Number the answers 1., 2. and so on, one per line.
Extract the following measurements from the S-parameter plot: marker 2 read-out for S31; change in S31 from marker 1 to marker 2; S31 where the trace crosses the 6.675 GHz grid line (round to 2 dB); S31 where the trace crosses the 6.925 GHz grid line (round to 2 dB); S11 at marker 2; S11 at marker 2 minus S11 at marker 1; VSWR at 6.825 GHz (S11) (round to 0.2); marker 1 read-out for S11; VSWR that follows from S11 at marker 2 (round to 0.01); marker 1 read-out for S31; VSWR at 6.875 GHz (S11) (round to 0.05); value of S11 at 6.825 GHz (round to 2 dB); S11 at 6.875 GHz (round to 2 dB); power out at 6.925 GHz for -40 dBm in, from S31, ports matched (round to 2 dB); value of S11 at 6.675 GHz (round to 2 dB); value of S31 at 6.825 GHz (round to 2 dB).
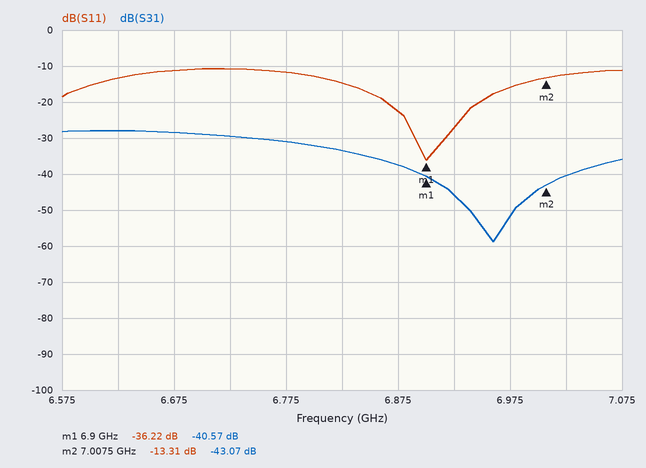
1. -43.07 dB
2. -2.50 dB
3. -28 dB
4. -46 dB
5. -13.31 dB
6. 22.91 dB
7. 1.4
8. -36.22 dB
9. 1.55
10. -40.57 dB
11. 1.15
12. -14 dB
13. -22 dB
14. -86 dBm
15. -12 dB
16. -34 dB
